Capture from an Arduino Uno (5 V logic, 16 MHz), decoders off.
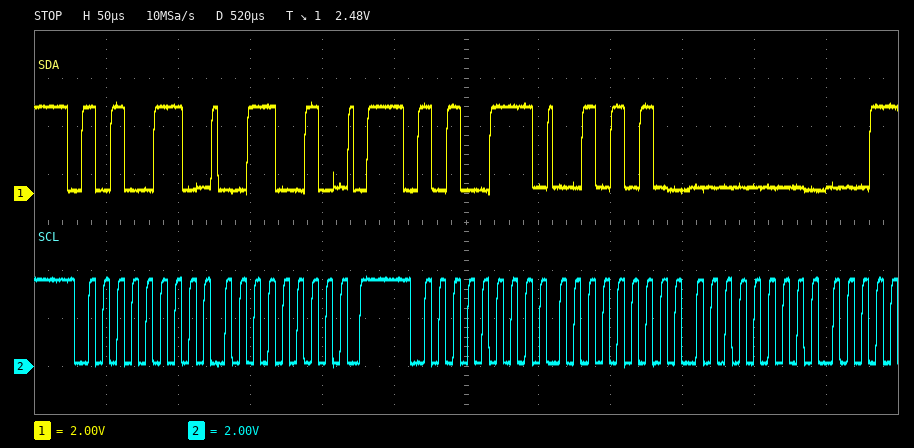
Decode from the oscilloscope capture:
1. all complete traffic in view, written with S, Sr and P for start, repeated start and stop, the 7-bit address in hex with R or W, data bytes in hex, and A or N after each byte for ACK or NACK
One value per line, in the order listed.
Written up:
S 53W A 32 A P S 53R A 2A A 00 A
